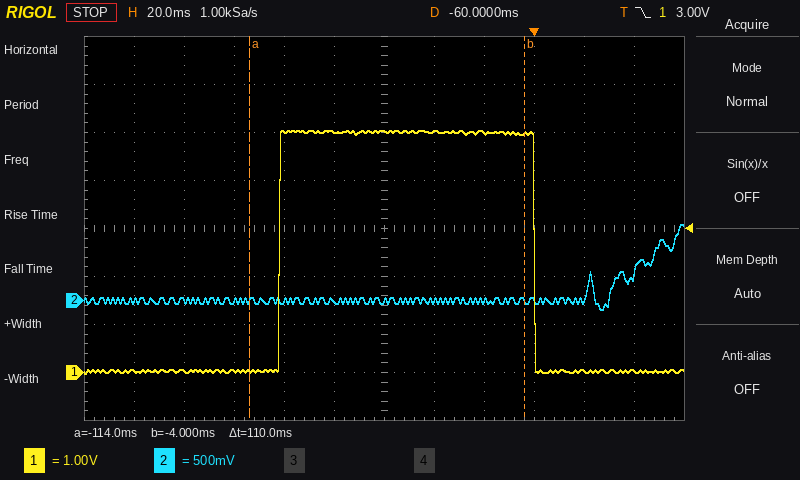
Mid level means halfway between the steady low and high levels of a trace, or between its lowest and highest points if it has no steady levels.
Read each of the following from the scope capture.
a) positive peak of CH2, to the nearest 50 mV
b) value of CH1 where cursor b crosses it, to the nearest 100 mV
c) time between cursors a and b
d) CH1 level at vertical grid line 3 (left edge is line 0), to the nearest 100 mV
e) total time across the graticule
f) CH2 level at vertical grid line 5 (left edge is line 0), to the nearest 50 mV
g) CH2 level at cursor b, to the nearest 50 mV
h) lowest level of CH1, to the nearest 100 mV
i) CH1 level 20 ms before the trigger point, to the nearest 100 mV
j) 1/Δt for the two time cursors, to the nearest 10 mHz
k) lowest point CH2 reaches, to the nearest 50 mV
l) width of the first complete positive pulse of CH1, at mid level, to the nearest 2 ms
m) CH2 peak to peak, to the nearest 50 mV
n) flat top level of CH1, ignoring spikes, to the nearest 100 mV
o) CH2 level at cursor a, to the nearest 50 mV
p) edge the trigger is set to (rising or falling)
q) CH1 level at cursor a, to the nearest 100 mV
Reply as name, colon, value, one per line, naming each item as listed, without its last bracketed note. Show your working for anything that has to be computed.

positive peak of CH2, to the nearest 50 mV: 800 mV
value of CH1 where cursor b crosses it, to the nearest 100 mV: 5.0 V
time between cursors a and b: 110 ms
CH1 level at vertical grid line 3 (left edge is line 0), to the nearest 100 mV: 0.0 V
total time across the graticule: 240 ms
CH2 level at vertical grid line 5 (left edge is line 0), to the nearest 50 mV: 0 mV
CH2 level at cursor b, to the nearest 50 mV: 0 mV
lowest level of CH1, to the nearest 100 mV: 0.0 V
CH1 level 20 ms before the trigger point, to the nearest 100 mV: 5.0 V
1/Δt for the two time cursors, to the nearest 10 mHz: 1 / 110 ms ≈ 9.09 Hz
lowest point CH2 reaches, to the nearest 50 mV: -100 mV
width of the first complete positive pulse of CH1, at mid level, to the nearest 2 ms: 102 ms
CH2 peak to peak, to the nearest 50 mV: 800 mV − (-100 mV) = 900 mV
flat top level of CH1, ignoring spikes, to the nearest 100 mV: 5.0 V
CH2 level at cursor a, to the nearest 50 mV: 0 mV
edge the trigger is set to: falling
CH1 level at cursor a, to the nearest 100 mV: 0.0 V
